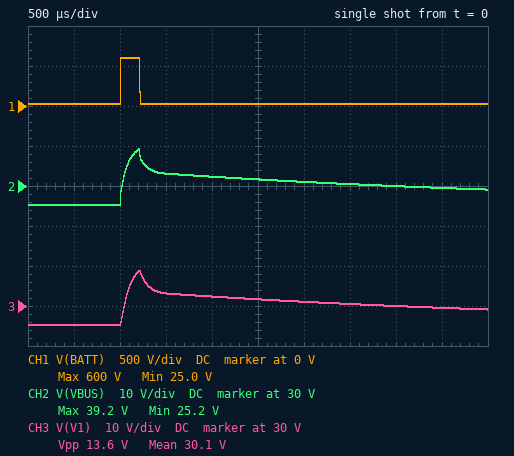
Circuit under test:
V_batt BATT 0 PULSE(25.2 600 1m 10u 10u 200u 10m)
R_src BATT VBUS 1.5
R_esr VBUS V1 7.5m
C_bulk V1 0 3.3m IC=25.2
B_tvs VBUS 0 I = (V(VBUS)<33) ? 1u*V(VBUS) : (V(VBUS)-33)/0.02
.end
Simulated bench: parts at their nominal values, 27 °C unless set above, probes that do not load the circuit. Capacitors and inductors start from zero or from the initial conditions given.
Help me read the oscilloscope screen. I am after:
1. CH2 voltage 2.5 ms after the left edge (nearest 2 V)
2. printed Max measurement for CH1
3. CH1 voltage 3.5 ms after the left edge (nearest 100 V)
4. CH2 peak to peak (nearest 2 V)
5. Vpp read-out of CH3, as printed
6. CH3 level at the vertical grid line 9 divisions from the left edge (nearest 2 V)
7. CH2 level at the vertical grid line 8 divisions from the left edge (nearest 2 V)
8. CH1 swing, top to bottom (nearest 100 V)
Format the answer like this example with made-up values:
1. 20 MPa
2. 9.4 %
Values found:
1. 32 V
2. 600 V
3. 0 V
4. 14 V
5. 13.6 V
6. 30 V
7. 30 V
8. 600 V
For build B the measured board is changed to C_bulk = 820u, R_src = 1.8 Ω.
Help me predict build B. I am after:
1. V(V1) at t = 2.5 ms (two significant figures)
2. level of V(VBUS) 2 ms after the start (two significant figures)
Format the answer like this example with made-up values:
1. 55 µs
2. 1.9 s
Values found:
1. 29 V
2. 30 V
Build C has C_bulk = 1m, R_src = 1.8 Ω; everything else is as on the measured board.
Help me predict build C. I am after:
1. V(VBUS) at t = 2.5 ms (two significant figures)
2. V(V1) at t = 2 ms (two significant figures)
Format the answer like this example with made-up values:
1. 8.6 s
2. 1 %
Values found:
1. 29 V
2. 31 V
